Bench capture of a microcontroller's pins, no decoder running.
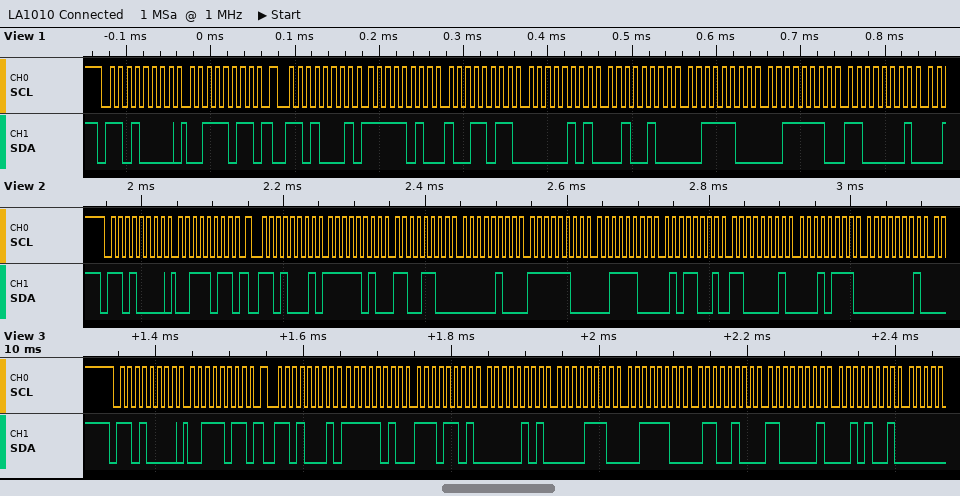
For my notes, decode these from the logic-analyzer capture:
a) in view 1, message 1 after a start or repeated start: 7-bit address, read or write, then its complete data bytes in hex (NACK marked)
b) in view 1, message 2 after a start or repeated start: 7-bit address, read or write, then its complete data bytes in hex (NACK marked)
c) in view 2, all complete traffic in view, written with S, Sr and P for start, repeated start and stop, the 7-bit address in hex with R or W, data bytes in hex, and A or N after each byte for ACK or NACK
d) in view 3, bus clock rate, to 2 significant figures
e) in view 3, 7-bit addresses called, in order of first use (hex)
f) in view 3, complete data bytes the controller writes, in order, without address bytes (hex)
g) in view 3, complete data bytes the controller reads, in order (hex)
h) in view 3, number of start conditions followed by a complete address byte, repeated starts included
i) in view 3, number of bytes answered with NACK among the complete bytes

0x68 write: 3B
0x68 read: FA 9B 05 24 3C 3E C1
S 68W A 3B A Sr 68R A FA A CC A 04 A FC A 3C A 59 A C1 A 17 A 01 A
100 kHz
0x68
3B
FA ED 05 0E 3C 64 C1 29
2
0
